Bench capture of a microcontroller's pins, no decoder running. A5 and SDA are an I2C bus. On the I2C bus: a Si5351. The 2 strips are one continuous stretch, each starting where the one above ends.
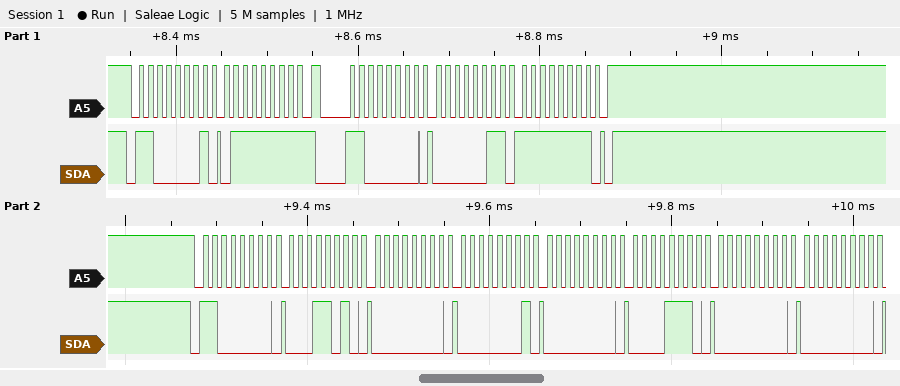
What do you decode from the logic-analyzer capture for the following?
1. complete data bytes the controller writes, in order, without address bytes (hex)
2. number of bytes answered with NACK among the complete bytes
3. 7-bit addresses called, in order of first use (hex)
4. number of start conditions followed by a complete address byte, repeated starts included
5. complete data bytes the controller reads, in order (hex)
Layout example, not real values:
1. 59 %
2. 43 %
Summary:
1. 03 FF 1A 00 01 00 0E 00 00
2. 1
3. 0x60
4. 3
5. 7F
